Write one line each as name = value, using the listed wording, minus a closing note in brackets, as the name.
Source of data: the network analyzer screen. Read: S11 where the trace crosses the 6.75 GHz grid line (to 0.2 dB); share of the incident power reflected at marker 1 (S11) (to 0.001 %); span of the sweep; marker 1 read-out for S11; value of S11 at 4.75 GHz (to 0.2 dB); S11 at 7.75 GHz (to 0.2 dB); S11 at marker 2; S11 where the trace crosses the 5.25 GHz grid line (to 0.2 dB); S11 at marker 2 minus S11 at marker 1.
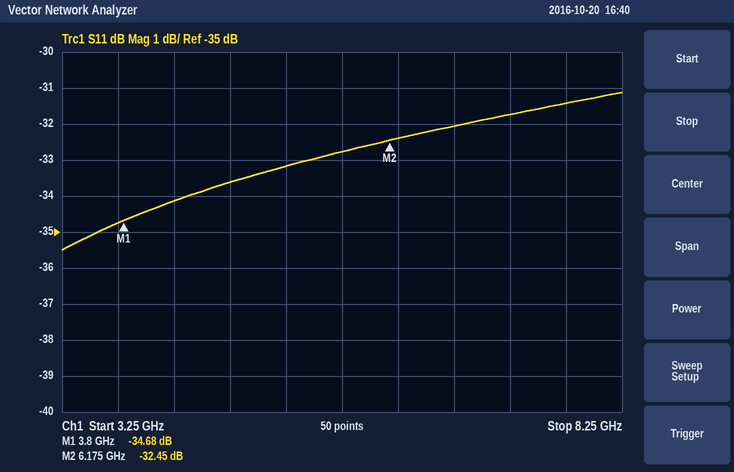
S11 where the trace crosses the 6.75 GHz grid line = -32.0 dB
share of the incident power reflected at marker 1 (S11) = 0.034 %
span of the sweep = 5 GHz
marker 1 read-out for S11 = -34.68 dB
value of S11 at 4.75 GHz = -33.6 dB
S11 at 7.75 GHz = -31.4 dB
S11 at marker 2 = -32.45 dB
S11 where the trace crosses the 5.25 GHz grid line = -33.2 dB
S11 at marker 2 minus S11 at marker 1 = 2.23 dB
